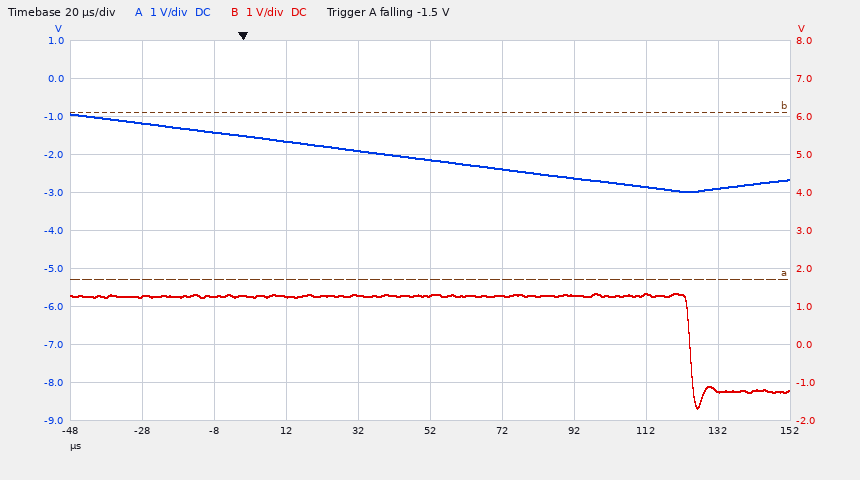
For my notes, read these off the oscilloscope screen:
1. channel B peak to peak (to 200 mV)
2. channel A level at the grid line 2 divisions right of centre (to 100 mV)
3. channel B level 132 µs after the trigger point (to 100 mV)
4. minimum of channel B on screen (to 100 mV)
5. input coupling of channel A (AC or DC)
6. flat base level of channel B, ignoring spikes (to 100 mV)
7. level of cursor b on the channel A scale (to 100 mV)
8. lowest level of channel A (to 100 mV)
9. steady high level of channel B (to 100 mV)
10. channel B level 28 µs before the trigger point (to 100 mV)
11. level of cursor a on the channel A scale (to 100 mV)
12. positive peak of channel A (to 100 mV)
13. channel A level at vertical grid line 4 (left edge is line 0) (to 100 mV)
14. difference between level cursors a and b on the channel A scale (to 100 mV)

3.0 V
-2.6 V
-1.2 V
-1.7 V
DC
-1.2 V
-900 mV
-3.0 V
1.3 V
1.3 V
-5.3 V
-900 mV
-1.9 V
4.4 V
